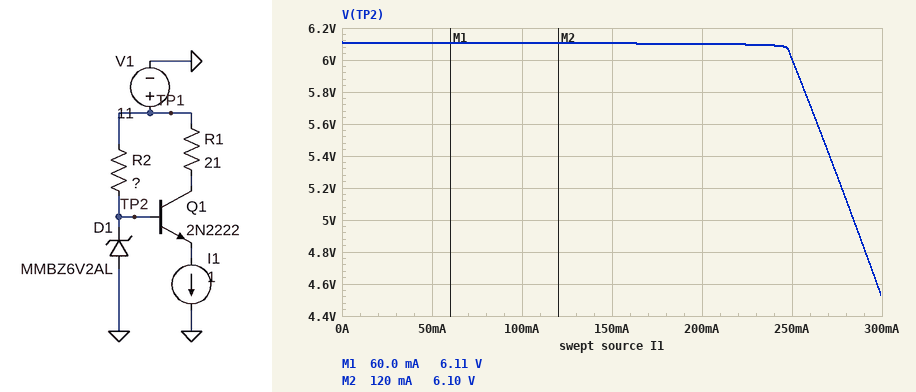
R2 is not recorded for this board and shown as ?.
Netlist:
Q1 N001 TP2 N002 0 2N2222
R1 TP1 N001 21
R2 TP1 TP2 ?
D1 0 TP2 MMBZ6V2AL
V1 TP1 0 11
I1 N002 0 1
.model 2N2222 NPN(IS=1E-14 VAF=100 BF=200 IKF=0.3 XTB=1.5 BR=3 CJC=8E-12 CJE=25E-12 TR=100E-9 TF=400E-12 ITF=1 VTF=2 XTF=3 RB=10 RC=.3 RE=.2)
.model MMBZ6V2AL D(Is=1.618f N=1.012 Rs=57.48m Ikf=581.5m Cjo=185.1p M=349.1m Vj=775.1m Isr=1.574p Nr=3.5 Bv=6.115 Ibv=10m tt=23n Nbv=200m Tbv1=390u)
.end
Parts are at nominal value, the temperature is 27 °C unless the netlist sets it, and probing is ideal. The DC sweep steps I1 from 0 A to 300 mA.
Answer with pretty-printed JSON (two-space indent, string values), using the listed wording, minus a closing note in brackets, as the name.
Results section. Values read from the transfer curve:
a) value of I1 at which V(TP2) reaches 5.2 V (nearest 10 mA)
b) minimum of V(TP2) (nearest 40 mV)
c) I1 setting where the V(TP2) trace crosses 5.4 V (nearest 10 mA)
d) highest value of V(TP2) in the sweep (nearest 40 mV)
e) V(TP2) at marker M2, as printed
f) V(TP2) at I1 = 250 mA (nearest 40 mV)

{
  "value of I1 at which V(TP2) reaches 5.2 V": "280 mA",
  "minimum of V(TP2)": "4.52 V",
  "I1 setting where the V(TP2) trace crosses 5.4 V": "270 mA",
  "highest value of V(TP2) in the sweep": "6.12 V",
  "V(TP2) at marker M2, as printed": "6.10 V",
  "V(TP2) at I1 = 250 mA": "6.00 V"
}
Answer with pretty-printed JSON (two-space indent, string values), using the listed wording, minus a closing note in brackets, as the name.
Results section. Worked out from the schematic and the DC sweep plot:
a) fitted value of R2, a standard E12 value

{
  "fitted value of R2, a standard E12 value": "2.2 kΩ"
}
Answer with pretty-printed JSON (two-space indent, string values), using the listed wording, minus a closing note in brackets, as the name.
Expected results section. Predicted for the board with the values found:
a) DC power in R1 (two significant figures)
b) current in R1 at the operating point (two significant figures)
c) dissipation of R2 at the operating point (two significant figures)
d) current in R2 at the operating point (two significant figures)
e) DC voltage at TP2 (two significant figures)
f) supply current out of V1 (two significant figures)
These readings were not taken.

{
  "DC power in R1": "11 W",
  "current in R1 at the operating point": "730 mA",
  "dissipation of R2 at the operating point": "64 mW",
  "current in R2 at the operating point": "5.4 mA",
  "DC voltage at TP2": "-890 mV",
  "supply current out of V1": "730 mA"
}
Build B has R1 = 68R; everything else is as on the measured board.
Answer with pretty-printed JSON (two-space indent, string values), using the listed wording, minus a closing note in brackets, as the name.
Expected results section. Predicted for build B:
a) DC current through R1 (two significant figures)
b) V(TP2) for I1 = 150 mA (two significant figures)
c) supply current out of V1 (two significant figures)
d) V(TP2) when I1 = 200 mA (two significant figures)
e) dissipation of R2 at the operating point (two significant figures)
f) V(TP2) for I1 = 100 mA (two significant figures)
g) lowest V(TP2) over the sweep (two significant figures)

{
  "DC current through R1": "290 mA",
  "V(TP2) for I1 = 150 mA": "1.8 V",
  "supply current out of V1": "300 mA",
  "V(TP2) when I1 = 200 mA": "-770 mV",
  "dissipation of R2 at the operating point": "65 mW",
  "V(TP2) for I1 = 100 mA": "5.1 V",
  "lowest V(TP2) over the sweep": "-850 mV"
}
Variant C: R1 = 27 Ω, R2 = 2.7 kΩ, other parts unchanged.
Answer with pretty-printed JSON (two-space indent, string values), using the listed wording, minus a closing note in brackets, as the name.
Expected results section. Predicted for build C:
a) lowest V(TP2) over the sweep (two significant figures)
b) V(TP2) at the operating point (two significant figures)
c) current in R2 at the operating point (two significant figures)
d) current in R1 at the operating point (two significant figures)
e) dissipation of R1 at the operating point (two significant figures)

{
  "lowest V(TP2) over the sweep": "3.0 V",
  "V(TP2) at the operating point": "-910 mV",
  "current in R2 at the operating point": "4.4 mA",
  "current in R1 at the operating point": "610 mA",
  "dissipation of R1 at the operating point": "10 W"
}
